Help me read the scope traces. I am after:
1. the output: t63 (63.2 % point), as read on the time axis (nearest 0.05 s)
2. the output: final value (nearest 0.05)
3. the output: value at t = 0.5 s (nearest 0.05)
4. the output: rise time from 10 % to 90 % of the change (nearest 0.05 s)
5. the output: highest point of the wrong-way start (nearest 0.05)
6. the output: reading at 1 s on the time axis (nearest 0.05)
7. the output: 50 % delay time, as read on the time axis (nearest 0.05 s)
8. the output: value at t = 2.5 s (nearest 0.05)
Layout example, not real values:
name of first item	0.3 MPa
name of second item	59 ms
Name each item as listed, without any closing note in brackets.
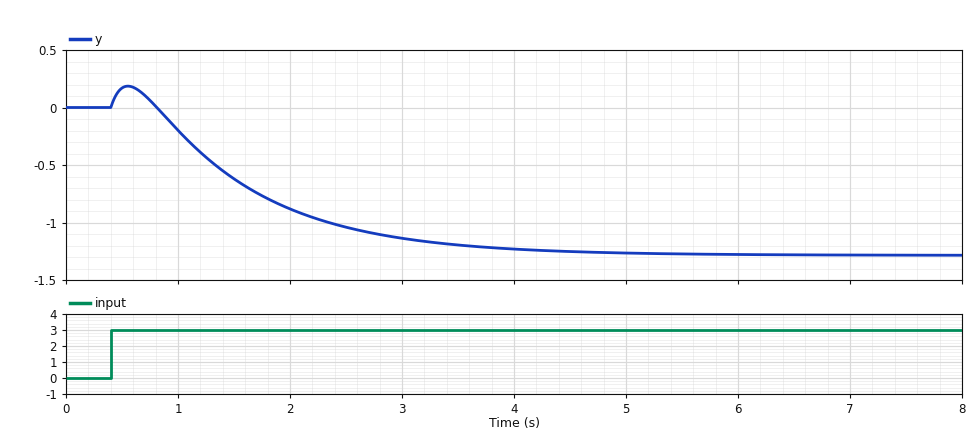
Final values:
the output: t63 (63.2 % point), as read on the time axis	1.85 s
the output: final value	-1.30
the output: value at t = 0.5 s	0.15
the output: rise time from 10 % to 90 % of the change	2.20 s
the output: highest point of the wrong-way start	0.20
the output: reading at 1 s on the time axis	-0.20
the output: 50 % delay time, as read on the time axis	1.55 s
the output: value at t = 2.5 s	-1.05
